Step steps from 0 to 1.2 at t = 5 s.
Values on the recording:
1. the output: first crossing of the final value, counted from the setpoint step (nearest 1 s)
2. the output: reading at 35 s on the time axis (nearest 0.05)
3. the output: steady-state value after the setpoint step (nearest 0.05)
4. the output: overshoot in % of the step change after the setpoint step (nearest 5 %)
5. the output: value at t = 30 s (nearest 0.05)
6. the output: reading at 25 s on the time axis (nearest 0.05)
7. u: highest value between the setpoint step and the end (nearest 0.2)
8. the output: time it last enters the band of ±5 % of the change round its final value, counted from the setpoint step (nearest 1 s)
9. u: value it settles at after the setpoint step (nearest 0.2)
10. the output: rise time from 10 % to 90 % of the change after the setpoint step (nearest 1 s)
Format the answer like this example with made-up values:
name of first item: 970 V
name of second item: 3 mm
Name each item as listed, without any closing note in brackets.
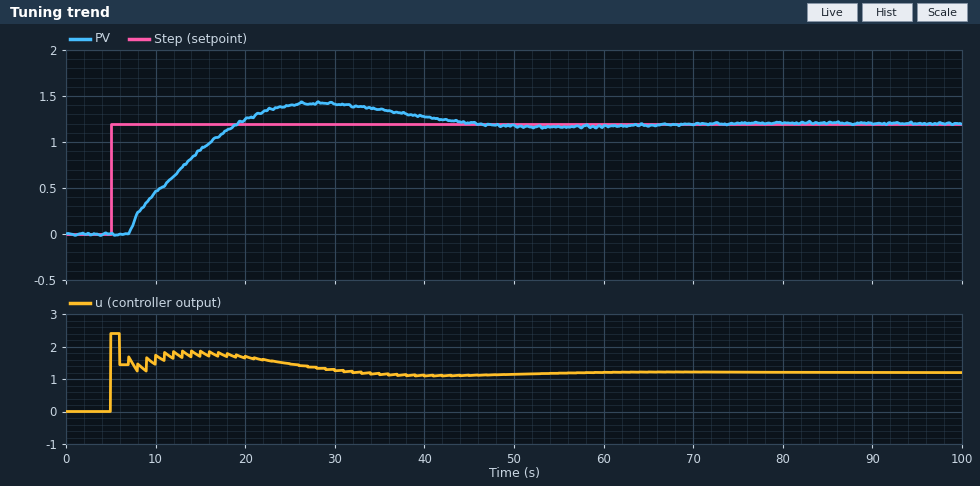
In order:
the output: first crossing of the final value, counted from the setpoint step: 14 s
the output: reading at 35 s on the time axis: 1.35
the output: steady-state value after the setpoint step: 1.20
the output: overshoot in % of the step change after the setpoint step: 20 %
the output: value at t = 30 s: 1.40
the output: reading at 25 s on the time axis: 1.40
u: highest value between the setpoint step and the end: 2.4
the output: time it last enters the band of ±5 % of the change round its final value, counted from the setpoint step: 36 s
u: value it settles at after the setpoint step: 1.2
the output: rise time from 10 % to 90 % of the change after the setpoint step: 10 s
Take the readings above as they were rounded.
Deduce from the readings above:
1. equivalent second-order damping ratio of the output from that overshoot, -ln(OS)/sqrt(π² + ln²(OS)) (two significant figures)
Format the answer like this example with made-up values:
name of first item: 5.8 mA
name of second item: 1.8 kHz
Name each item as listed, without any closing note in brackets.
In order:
equivalent second-order damping ratio of the output from that overshoot, -ln(OS)/sqrt(π² + ln²(OS)): 0.46
